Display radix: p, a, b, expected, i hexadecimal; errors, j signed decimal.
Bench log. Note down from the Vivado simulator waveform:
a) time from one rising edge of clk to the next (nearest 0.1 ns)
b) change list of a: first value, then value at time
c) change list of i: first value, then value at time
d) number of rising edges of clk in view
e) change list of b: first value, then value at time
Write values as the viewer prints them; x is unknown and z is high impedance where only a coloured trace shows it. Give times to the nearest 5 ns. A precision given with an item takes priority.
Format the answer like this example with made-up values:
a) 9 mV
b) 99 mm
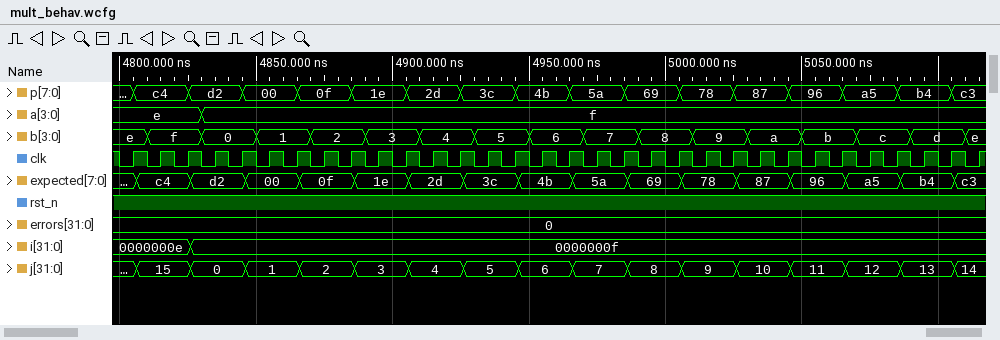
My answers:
a) 10 ns
b) e, f at 4830 ns
c) 0000000e, 0000000f at 4825 ns
d) 32
e) e, f at 4810 ns, 0 at 4830 ns, 1 at 4850 ns, 2 at 4870 ns, 3 at 4890 ns, 4 at 4910 ns, 5 at 4930 ns, 6 at 4950 ns, 7 at 4970 ns, 8 at 4990 ns, 9 at 5010 ns, a at 5030 ns, b at 5050 ns, c at 5070 ns, d at 5090 ns, e at 5110 ns
